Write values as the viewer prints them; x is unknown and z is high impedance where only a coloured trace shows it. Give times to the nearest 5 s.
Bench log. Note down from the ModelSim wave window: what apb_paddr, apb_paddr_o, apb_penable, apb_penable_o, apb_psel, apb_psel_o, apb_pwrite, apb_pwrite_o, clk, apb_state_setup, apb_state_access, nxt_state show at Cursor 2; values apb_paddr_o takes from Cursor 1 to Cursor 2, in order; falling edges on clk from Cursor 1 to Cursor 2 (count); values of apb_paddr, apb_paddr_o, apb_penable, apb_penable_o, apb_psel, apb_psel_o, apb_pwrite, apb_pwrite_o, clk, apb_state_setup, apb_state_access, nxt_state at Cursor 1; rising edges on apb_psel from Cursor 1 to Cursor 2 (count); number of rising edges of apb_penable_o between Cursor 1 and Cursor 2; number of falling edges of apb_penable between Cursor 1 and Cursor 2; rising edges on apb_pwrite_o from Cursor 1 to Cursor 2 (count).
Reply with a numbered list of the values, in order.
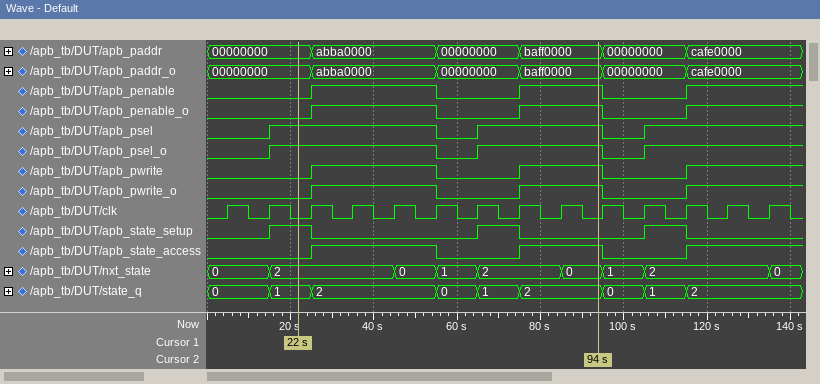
1. apb_paddr=baff0000, apb_paddr_o=baff0000, apb_penable=1, apb_penable_o=1, apb_psel=1, apb_psel_o=1, apb_pwrite=1, apb_pwrite_o=1, clk=0, apb_state_setup=0, apb_state_access=1, nxt_state=0
2. 00000000, abba0000, 00000000, baff0000
3. 7
4. apb_paddr=00000000, apb_paddr_o=00000000, apb_penable=0, apb_penable_o=0, apb_psel=1, apb_psel_o=1, apb_pwrite=0, apb_pwrite_o=0, clk=0, apb_state_setup=1, apb_state_access=0, nxt_state=2
5. 1
6. 2
7. 1
8. 2
